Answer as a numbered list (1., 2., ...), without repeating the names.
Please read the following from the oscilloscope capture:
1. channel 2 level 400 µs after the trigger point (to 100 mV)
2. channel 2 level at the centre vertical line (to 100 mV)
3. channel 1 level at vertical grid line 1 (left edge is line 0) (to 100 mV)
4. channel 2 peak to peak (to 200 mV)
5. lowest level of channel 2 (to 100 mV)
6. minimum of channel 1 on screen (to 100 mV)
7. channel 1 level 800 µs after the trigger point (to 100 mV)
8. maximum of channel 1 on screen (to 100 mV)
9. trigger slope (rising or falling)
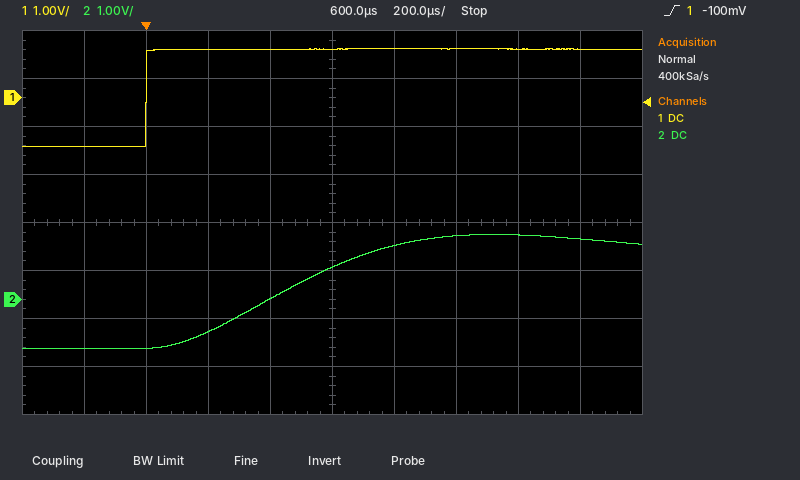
1. 0.0 V
2. 700 mV
3. -1.0 V
4. 2.4 V
5. -1.0 V
6. -1.0 V
7. 1.0 V
8. 1.0 V
9. rising
